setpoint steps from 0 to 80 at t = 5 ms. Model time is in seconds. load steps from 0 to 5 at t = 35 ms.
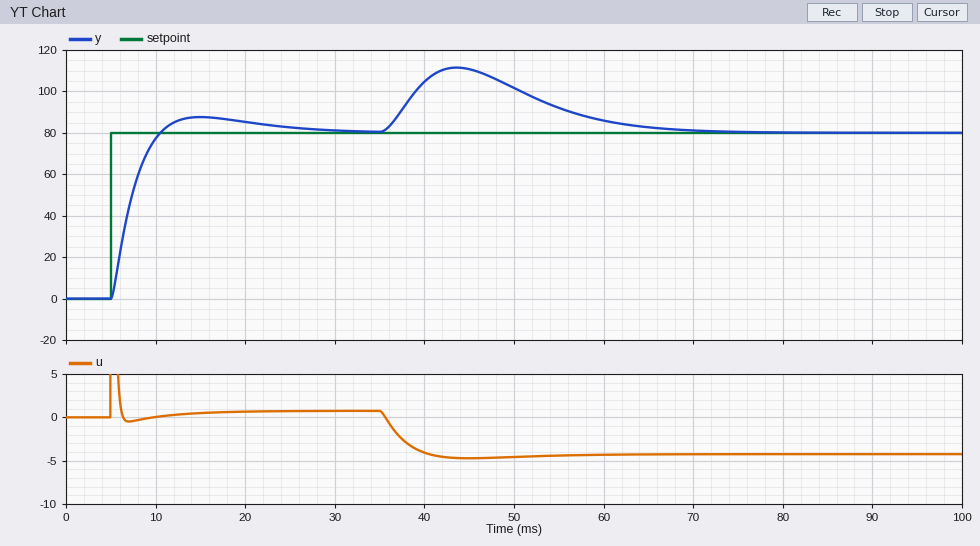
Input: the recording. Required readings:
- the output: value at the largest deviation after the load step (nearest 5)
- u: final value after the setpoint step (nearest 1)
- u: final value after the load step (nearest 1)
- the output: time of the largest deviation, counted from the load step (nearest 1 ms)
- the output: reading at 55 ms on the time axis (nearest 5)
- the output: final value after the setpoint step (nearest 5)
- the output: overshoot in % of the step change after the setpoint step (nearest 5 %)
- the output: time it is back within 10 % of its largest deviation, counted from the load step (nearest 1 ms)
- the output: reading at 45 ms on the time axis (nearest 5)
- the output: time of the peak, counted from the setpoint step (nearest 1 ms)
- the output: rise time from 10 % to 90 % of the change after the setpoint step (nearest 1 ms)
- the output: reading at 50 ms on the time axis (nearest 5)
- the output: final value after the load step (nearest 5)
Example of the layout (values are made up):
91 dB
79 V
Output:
110
1
-4
9 ms
90
80
10 %
29 ms
110
10 ms
4 ms
100
80
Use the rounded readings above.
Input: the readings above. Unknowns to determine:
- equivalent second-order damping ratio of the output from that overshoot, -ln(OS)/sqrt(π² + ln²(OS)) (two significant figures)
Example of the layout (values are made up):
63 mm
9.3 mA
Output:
0.59
